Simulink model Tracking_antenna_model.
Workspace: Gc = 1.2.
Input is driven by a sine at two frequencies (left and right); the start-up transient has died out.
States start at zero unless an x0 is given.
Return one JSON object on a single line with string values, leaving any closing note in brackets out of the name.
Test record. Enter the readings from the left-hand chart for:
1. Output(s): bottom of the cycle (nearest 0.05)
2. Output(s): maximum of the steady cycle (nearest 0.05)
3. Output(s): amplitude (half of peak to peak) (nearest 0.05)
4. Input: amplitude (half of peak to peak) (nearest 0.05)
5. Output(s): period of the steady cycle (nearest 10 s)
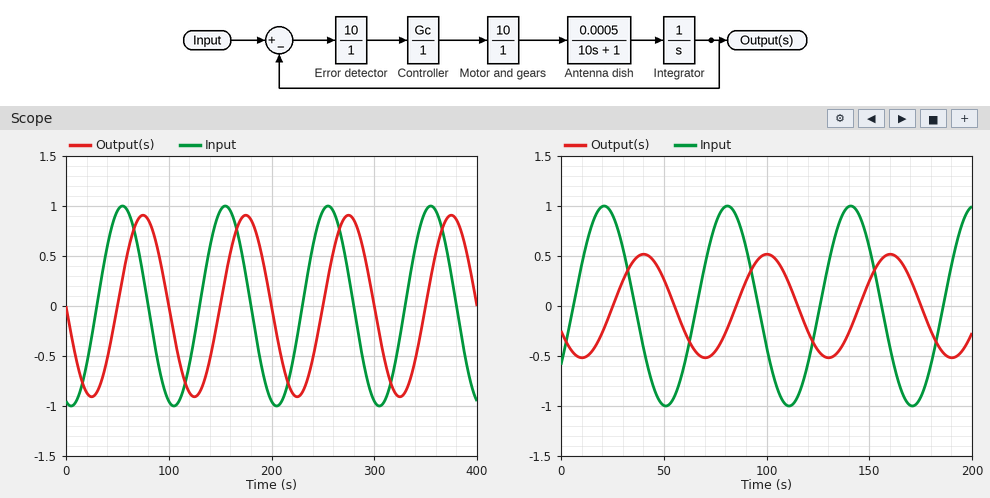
{"Output(s): bottom of the cycle": "-0.90", "Output(s): maximum of the steady cycle": "0.90", "Output(s): amplitude (half of peak to peak)": "0.90", "Input: amplitude (half of peak to peak)": "1.00", "Output(s): period of the steady cycle": "100 s"}
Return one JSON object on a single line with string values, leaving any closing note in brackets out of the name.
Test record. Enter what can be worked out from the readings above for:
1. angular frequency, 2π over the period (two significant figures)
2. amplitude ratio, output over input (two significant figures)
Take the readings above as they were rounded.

{"angular frequency, 2π over the period": "0.063 rad/s", "amplitude ratio, output over input": "0.90"}
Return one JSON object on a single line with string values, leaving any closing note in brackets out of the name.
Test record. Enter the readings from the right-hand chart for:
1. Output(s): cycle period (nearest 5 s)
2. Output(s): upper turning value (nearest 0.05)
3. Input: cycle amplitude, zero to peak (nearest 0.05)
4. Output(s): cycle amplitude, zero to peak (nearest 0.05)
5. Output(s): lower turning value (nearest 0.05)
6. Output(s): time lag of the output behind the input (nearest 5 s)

{"Output(s): cycle period": "60 s", "Output(s): upper turning value": "0.50", "Input: cycle amplitude, zero to peak": "1.00", "Output(s): cycle amplitude, zero to peak": "0.50", "Output(s): lower turning value": "-0.50", "Output(s): time lag of the output behind the input": "20 s"}
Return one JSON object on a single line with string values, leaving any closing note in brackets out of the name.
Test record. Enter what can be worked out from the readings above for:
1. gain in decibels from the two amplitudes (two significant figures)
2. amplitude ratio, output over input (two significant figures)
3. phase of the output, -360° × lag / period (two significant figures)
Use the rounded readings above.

{"gain in decibels from the two amplitudes": "-6.0 dB", "amplitude ratio, output over input": "0.50", "phase of the output, -360° × lag / period": "-120°"}
